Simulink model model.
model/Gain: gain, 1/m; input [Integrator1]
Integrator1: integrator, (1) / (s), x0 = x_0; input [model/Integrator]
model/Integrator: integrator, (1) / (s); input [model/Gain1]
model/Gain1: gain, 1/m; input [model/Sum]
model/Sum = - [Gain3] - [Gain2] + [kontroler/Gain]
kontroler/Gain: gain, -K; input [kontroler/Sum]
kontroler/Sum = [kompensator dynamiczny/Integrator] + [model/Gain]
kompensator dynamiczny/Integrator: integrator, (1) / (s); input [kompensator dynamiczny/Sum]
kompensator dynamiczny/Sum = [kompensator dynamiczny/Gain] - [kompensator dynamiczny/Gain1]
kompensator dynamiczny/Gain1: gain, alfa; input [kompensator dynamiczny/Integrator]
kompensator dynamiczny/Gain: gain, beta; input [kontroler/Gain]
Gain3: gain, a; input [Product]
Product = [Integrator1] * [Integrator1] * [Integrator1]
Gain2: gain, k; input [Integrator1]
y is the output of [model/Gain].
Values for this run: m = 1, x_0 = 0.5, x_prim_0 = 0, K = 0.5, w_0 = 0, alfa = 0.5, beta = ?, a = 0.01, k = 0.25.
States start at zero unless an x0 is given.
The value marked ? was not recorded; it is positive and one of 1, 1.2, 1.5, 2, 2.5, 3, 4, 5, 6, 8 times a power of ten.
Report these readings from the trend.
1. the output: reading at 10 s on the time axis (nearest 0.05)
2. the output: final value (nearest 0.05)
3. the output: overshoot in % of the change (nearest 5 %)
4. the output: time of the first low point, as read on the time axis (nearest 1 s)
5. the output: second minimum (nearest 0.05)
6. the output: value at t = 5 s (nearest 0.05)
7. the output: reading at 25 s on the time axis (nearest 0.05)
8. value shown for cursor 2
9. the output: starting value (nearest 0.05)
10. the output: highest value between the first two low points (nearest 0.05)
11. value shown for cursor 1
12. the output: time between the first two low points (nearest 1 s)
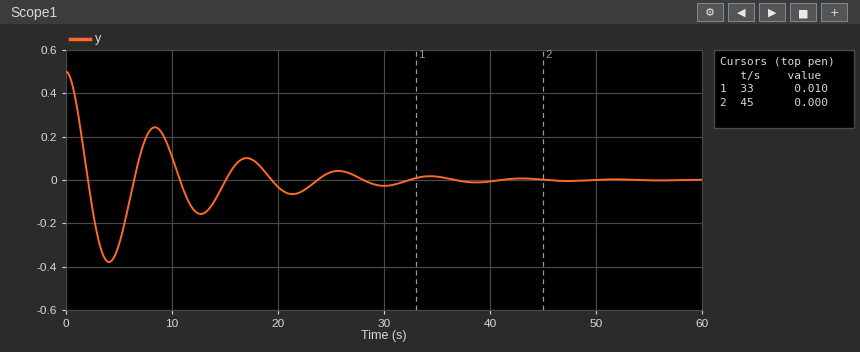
0.10
0.00
75 %
4 s
-0.15
-0.30
0.05
0.000
0.50
0.25
0.010
9 s
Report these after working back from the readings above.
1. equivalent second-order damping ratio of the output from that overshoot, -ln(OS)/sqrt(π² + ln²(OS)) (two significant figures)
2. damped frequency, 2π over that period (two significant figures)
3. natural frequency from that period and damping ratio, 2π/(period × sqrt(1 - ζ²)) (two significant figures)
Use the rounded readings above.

0.091
0.70 rad/s
0.70 rad/s
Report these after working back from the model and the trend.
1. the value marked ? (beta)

1.5
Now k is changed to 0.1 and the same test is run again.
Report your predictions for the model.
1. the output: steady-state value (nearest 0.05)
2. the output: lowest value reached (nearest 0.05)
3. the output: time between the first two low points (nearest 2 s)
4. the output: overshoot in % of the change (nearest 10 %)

0.00
-0.35
10 s
70 %
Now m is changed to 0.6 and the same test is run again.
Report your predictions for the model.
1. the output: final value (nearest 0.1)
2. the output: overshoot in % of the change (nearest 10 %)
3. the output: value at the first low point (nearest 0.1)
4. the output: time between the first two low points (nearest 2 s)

0.0
70 %
-0.6
6 s
